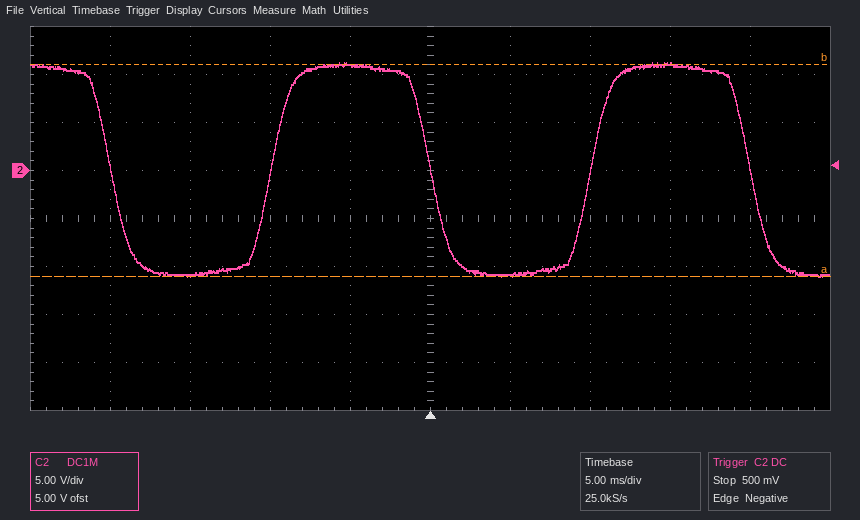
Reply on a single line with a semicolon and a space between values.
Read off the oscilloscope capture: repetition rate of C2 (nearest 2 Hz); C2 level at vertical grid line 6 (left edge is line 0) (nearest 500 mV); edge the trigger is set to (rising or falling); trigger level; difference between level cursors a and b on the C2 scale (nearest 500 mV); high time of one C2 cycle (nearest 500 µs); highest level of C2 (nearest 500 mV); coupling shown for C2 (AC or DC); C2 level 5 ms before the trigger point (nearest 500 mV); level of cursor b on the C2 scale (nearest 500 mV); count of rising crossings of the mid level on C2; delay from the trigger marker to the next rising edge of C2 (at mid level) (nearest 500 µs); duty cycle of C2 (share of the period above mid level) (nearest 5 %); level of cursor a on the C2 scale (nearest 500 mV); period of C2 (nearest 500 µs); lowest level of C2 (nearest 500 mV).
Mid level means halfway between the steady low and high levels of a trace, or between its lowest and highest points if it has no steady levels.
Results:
50 Hz; -11.0 V; falling; 500 mV; 22.0 V; 10.0 ms; 11.0 V; DC; 11.0 V; 11.0 V; 2; 10.0 ms; 50 %; -11.0 V; 20.0 ms; -11.0 V
